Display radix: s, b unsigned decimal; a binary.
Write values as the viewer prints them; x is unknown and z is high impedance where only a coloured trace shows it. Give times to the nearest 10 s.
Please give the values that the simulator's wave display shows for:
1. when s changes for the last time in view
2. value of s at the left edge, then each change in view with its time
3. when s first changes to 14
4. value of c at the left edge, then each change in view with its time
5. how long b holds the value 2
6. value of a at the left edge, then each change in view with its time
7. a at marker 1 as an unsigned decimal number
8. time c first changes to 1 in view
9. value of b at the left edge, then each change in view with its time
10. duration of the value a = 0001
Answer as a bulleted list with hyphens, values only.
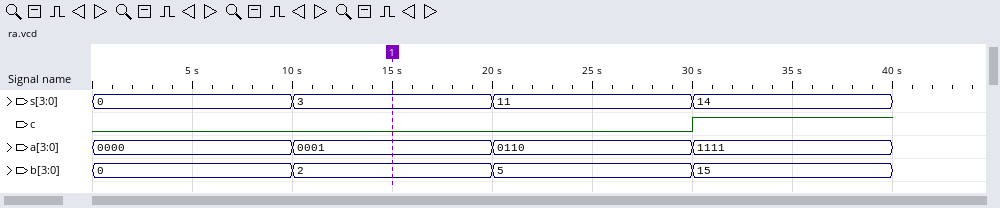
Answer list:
- 30 s
- 0, 3 at 10 s, 11 at 20 s, 14 at 30 s
- 30 s
- 0, 1 at 30 s
- 10 s
- 0000, 0001 at 10 s, 0110 at 20 s, 1111 at 30 s
- 1
- 30 s
- 0, 2 at 10 s, 5 at 20 s, 15 at 30 s
- 10 s
